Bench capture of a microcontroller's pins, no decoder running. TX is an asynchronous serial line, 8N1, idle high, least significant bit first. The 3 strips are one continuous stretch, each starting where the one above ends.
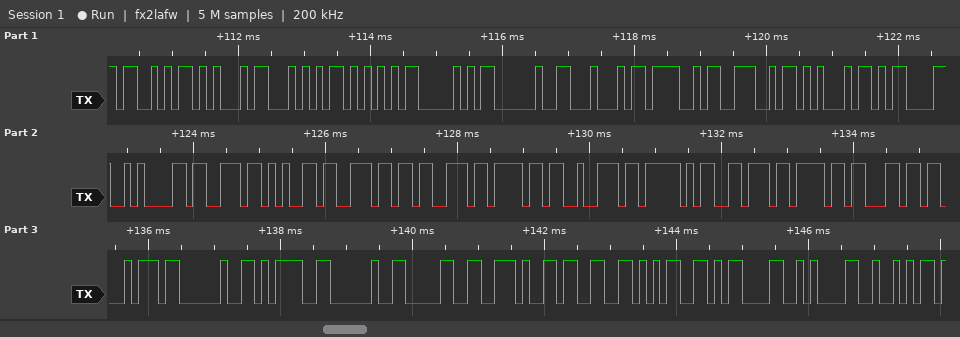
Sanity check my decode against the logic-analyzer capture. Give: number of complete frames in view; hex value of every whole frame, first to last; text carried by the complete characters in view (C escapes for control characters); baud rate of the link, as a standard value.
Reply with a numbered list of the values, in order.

1. 33
2. 53 45 54 55 50 20 44 4F 4E 45 0D 0A 73 65 6E 73 6F 72 5F 76 6F 6C 74 20 3D 20 30 2E 33 35 0D 0A 52
3. "SETUP DONE\r\nsensor_volt = 0.35\r\nR"
4. 9600 baud
